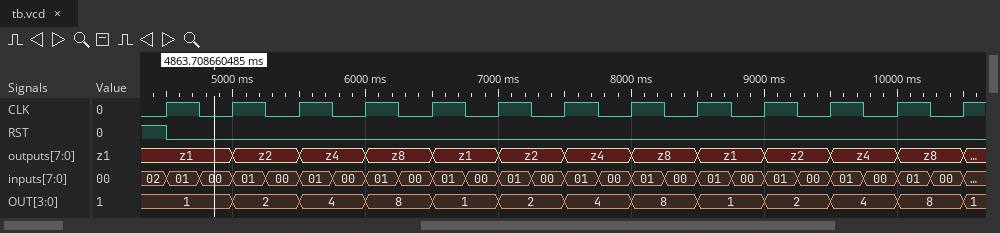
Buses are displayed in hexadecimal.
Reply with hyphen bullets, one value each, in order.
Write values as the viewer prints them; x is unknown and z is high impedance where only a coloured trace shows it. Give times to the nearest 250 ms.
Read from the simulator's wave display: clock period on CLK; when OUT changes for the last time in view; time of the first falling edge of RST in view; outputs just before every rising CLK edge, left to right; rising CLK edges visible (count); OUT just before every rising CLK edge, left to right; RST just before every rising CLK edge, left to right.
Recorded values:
- 500 ms
- 10500 ms
- 4500 ms
- z1, z1, z2, z4, z8, z1, z2, z4, z8, z1, z2, z4, z8
- 13
- 1, 1, 2, 4, 8, 1, 2, 4, 8, 1, 2, 4, 8
- 1 0 0 0 0 0 0 0 0 0 0 0 0
